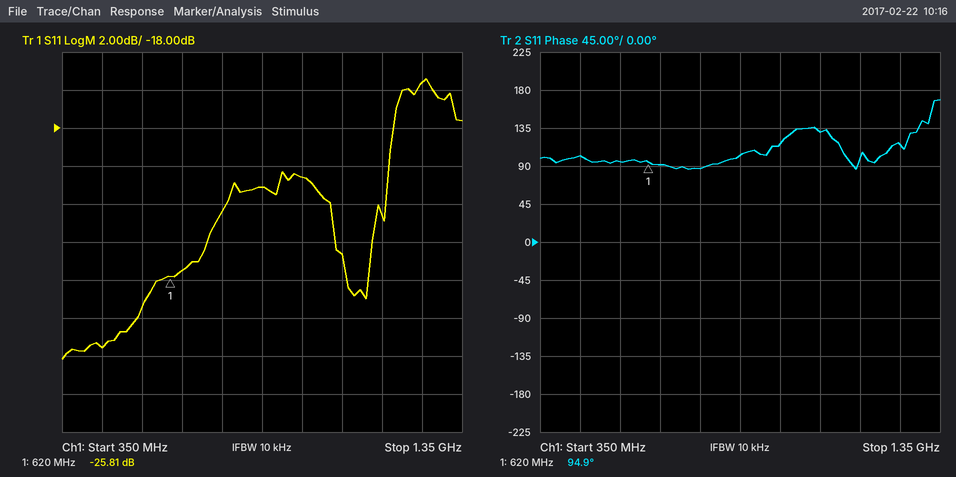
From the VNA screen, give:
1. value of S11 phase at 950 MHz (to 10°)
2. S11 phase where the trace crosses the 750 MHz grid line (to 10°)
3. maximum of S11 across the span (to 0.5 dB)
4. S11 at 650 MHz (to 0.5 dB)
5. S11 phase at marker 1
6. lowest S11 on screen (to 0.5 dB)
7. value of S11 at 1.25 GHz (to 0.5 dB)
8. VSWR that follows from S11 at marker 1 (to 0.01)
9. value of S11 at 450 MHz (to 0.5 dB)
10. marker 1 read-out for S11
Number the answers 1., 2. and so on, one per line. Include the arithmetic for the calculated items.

1. 120°
2. 90°
3. -15.5 dB
4. -25.5 dB
5. 94.9°
6. -30.0 dB
7. -15.5 dB
8. (1 + 0.0512)/(1 − 0.0512) ≈ 1.11
9. -29.5 dB
10. -25.81 dB
